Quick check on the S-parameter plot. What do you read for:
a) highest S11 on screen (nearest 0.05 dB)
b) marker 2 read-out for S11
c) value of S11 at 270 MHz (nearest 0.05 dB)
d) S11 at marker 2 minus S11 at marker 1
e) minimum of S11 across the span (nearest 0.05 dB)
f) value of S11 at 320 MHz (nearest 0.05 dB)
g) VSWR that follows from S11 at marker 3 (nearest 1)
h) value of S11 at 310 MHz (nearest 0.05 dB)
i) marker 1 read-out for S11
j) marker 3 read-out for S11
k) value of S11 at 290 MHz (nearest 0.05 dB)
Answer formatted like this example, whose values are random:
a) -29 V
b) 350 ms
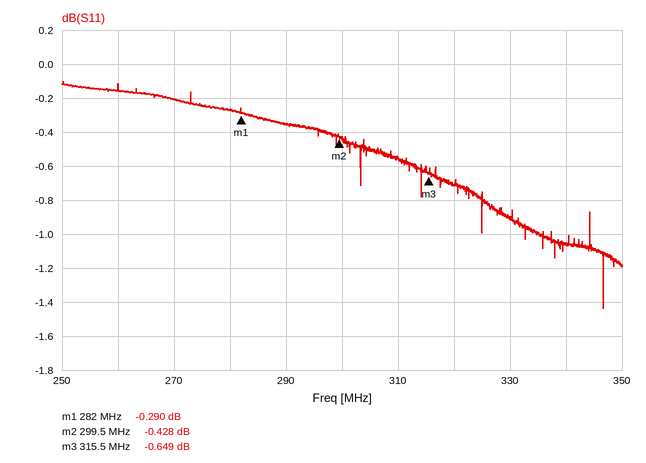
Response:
a) -0.10 dB
b) -0.428 dB
c) -0.20 dB
d) -0.138 dB
e) -1.45 dB
f) -0.70 dB
g) 27
h) -0.55 dB
i) -0.290 dB
j) -0.649 dB
k) -0.35 dB
